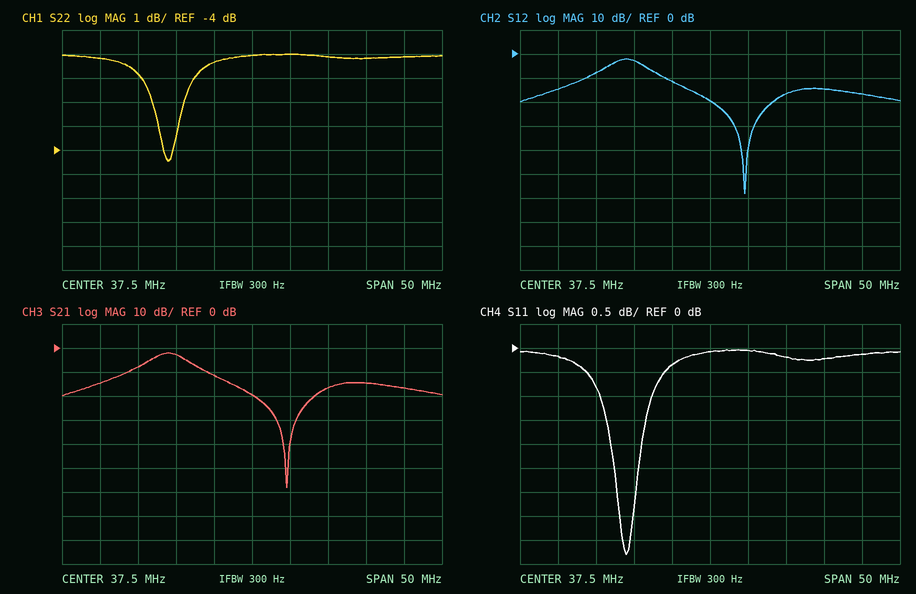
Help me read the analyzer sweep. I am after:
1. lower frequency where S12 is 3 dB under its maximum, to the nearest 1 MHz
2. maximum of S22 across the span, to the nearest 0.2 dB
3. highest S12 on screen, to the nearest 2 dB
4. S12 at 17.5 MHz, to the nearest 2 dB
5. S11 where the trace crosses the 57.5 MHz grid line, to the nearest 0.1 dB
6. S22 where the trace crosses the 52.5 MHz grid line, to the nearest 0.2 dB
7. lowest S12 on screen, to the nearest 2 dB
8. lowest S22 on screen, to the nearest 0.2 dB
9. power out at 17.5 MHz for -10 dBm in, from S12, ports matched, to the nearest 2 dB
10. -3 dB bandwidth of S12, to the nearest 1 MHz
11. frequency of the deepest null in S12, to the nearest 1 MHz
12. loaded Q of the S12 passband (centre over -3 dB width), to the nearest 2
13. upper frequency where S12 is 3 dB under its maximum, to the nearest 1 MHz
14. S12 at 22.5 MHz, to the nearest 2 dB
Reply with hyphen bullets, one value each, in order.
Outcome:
- 24 MHz
- 0.0 dB
- -2 dB
- -14 dB
- -0.1 dB
- -0.2 dB
- -58 dB
- -4.4 dB
- -24 dBm
- 5 MHz
- 42 MHz
- 6
- 29 MHz
- -8 dB
